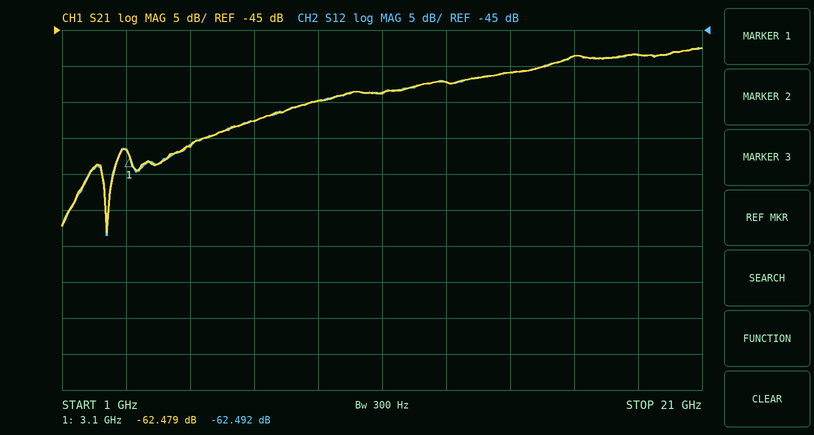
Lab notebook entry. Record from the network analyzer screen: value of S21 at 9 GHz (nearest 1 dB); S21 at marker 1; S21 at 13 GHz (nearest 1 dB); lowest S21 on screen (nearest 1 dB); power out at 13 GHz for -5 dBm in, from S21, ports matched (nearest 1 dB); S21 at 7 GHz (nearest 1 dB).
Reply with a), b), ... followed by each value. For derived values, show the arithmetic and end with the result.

a) -55 dB
b) -62.479 dB
c) -52 dB
d) -73 dB
e) -5 dBm + (-52 dB) = -57 dBm
f) -58 dB
